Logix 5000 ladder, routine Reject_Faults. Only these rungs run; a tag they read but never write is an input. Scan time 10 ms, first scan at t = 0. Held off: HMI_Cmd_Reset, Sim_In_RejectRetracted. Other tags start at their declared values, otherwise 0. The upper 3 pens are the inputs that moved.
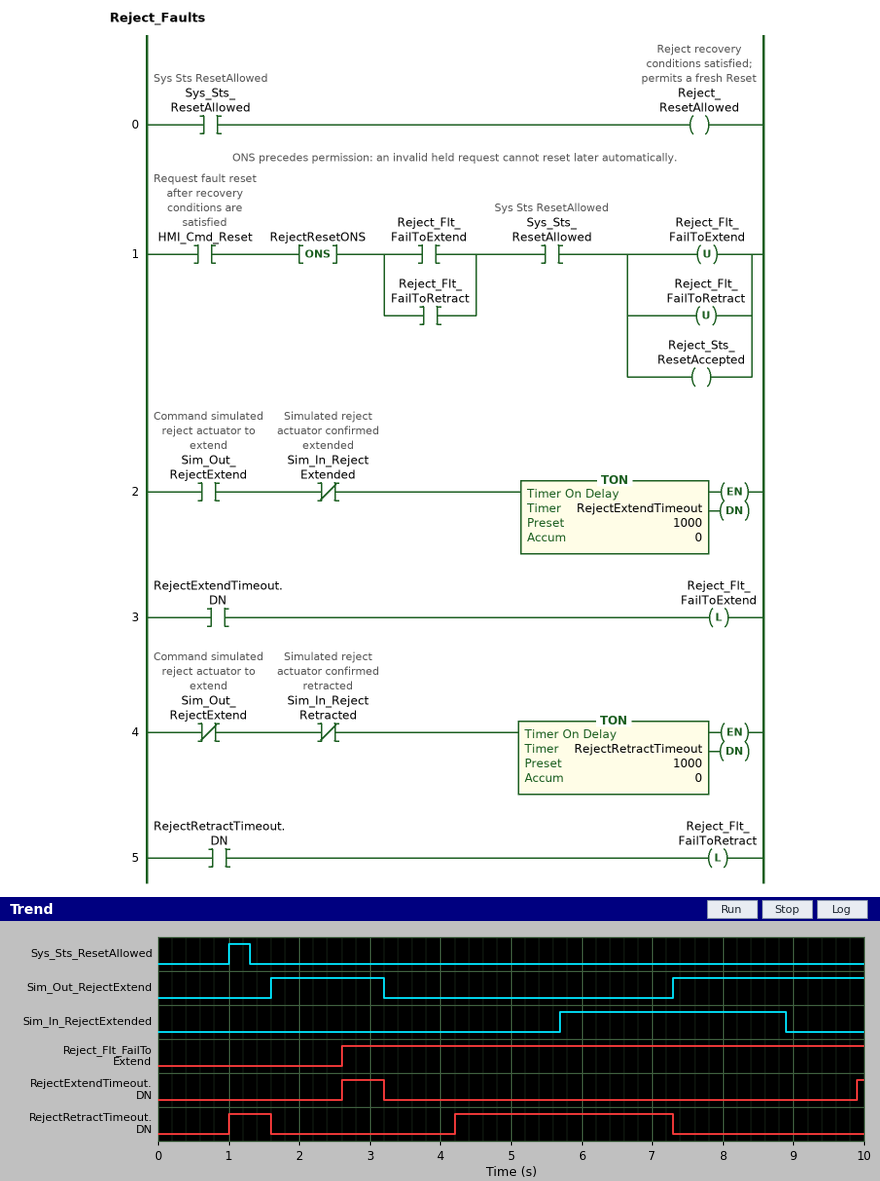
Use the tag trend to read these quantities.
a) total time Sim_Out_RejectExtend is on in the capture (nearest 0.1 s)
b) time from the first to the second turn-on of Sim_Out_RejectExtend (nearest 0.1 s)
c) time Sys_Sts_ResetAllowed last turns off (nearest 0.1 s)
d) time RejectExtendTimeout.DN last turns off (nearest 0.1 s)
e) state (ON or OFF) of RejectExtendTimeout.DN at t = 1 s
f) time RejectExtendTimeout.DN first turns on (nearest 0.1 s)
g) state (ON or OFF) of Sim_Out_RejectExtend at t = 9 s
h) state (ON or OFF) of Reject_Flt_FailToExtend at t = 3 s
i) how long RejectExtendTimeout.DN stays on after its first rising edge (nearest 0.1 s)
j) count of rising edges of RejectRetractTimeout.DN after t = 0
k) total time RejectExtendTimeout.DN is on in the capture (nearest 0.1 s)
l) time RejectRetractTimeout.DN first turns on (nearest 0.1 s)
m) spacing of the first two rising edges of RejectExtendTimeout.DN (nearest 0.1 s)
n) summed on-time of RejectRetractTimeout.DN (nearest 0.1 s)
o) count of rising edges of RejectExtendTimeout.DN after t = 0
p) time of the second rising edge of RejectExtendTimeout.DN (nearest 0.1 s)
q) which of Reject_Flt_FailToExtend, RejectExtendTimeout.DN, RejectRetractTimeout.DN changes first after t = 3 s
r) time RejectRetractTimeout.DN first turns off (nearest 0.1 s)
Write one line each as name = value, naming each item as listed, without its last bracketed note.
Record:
total time Sim_Out_RejectExtend is on in the capture = 4.3 s
time from the first to the second turn-on of Sim_Out_RejectExtend = 5.7 s
time Sys_Sts_ResetAllowed last turns off = 1.3 s
time RejectExtendTimeout.DN last turns off = 3.2 s
state (ON or OFF) of RejectExtendTimeout.DN at t = 1 s = OFF
time RejectExtendTimeout.DN first turns on = 2.6 s
state (ON or OFF) of Sim_Out_RejectExtend at t = 9 s = ON
state (ON or OFF) of Reject_Flt_FailToExtend at t = 3 s = ON
how long RejectExtendTimeout.DN stays on after its first rising edge = 0.6 s
count of rising edges of RejectRetractTimeout.DN after t = 0 = 2
total time RejectExtendTimeout.DN is on in the capture = 0.7 s
time RejectRetractTimeout.DN first turns on = 1.0 s
spacing of the first two rising edges of RejectExtendTimeout.DN = 7.3 s
summed on-time of RejectRetractTimeout.DN = 3.7 s
count of rising edges of RejectExtendTimeout.DN after t = 0 = 2
time of the second rising edge of RejectExtendTimeout.DN = 9.9 s
which of Reject_Flt_FailToExtend, RejectExtendTimeout.DN, RejectRetractTimeout.DN changes first after t = 3 s = RejectExtendTimeout.DN
time RejectRetractTimeout.DN first turns off = 1.6 s
